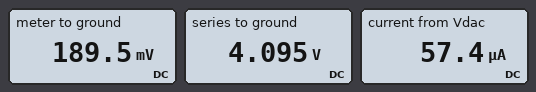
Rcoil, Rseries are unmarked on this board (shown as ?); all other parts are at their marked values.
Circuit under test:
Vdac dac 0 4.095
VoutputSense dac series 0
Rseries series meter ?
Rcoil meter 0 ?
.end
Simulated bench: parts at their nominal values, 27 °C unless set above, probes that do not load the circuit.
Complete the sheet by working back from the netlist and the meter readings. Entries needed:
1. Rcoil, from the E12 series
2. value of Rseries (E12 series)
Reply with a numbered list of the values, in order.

1. 3.3 kΩ
2. 68 kΩ
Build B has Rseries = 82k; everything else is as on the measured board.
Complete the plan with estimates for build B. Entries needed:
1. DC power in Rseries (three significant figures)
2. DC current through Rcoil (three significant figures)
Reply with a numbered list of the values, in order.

1. 189 µW
2. 48.0 µA
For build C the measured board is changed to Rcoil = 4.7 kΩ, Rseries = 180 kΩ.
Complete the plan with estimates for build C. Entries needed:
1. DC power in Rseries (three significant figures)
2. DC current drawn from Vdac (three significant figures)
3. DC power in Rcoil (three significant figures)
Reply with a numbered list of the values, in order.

1. 88.5 µW
2. 22.2 µA
3. 2.31 µW
